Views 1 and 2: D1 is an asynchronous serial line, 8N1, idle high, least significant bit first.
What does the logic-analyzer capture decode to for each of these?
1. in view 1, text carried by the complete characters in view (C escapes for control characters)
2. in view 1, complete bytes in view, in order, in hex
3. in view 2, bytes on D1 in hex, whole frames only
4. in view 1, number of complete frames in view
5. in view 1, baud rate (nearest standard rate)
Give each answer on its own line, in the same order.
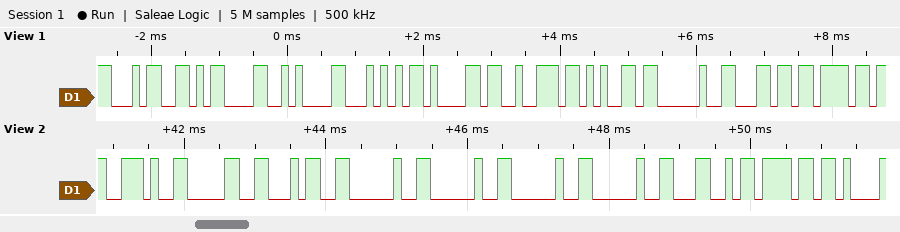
"4\r\nTare lo"
34 0D 0A 54 61 72 65 20 6C 6F
2E 30 34 20 20 20 20 4C 6F
10
9600 baud
